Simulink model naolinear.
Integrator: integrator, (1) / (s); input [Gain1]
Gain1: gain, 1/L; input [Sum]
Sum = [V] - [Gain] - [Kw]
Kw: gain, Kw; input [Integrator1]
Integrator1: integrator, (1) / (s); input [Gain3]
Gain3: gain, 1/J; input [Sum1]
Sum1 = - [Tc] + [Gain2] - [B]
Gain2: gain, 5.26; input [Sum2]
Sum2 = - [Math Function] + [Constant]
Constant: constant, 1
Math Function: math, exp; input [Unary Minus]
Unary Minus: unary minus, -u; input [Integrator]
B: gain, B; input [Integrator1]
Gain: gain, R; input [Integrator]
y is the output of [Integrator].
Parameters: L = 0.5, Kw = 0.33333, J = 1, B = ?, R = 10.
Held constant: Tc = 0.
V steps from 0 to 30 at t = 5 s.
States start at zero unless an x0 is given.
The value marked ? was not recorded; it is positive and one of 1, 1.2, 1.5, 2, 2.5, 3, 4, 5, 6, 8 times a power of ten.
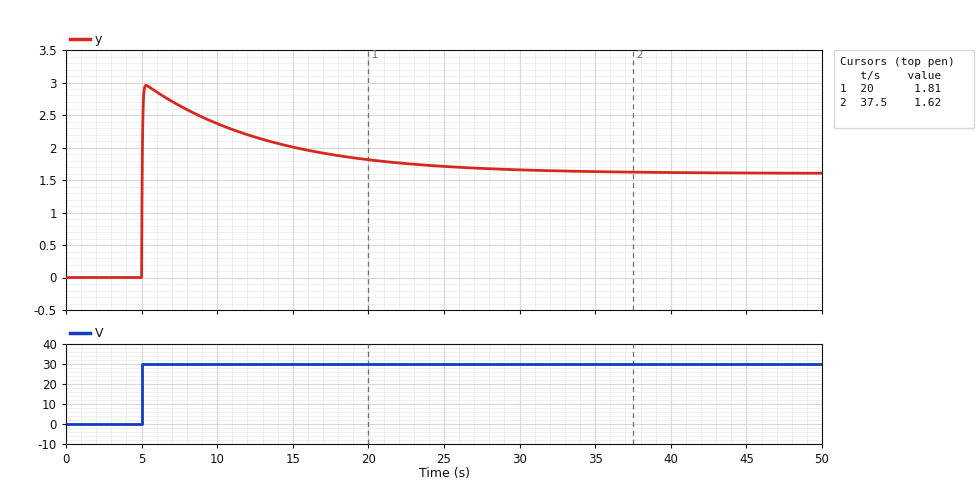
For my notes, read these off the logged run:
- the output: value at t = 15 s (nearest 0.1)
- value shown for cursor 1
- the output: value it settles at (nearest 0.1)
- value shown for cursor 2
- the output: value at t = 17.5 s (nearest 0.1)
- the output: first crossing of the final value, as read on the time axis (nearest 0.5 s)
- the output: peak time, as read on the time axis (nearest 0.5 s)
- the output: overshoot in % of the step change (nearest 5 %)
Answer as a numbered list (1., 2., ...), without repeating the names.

1. 2.0
2. 1.81
3. 1.6
4. 1.62
5. 1.9
6. 5.0 s
7. 5.5 s
8. 85 %
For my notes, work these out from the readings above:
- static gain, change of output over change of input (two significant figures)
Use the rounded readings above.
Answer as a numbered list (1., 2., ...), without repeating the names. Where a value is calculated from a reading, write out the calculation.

1. (1.6 - 0) / (30 - 0) = 0.053
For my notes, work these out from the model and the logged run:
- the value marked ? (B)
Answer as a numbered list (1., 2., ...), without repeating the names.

1. 0.1
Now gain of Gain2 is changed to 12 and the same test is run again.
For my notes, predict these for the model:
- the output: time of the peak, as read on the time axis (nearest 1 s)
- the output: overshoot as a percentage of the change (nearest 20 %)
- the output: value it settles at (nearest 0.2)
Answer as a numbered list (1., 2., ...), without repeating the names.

1. 5 s
2. 260 %
3. 0.8
